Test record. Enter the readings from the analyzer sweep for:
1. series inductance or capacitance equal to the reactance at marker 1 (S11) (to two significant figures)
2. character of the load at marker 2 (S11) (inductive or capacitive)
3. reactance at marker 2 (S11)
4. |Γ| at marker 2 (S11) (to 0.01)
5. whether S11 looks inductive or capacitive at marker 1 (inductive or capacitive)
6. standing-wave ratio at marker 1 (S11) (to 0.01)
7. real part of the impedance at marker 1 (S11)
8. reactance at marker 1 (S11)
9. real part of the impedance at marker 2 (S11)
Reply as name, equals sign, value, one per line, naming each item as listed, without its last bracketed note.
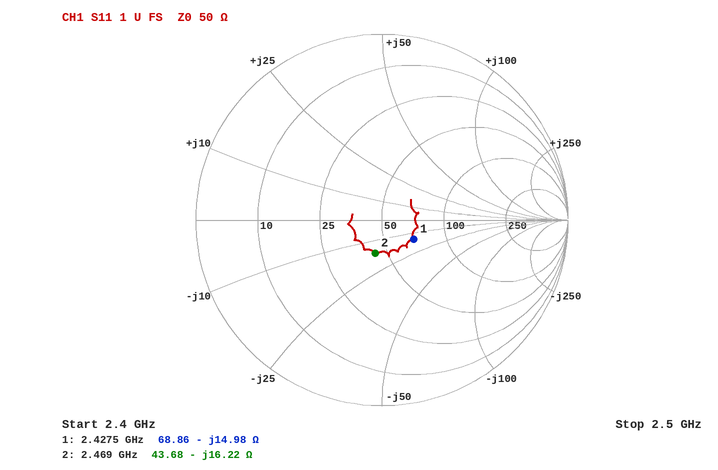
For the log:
series inductance or capacitance equal to the reactance at marker 1 (S11) = 4.4 pF
character of the load at marker 2 (S11) = capacitive
reactance at marker 2 = -16.22 Ω
|Γ| at marker 2 (S11) = 0.18
whether S11 looks inductive or capacitive at marker 1 = capacitive
standing-wave ratio at marker 1 (S11) = 1.50
real part of the impedance at marker 1 = 68.86 Ω
reactance at marker 1 = -14.98 Ω
real part of the impedance at marker 2 = 43.68 Ω
